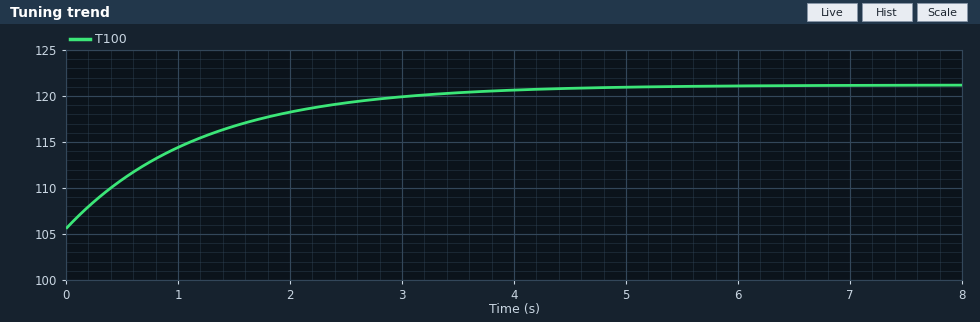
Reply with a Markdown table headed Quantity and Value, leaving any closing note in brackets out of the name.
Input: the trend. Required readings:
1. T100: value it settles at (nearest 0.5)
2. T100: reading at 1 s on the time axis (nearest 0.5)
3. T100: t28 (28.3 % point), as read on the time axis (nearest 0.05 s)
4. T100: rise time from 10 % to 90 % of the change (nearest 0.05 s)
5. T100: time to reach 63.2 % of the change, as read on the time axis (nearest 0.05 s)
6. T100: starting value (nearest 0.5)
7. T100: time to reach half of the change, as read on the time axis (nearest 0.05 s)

| Quantity | Value |
|---|---|
| T100: value it settles at | 121.0 |
| T100: reading at 1 s on the time axis | 114.5 |
| T100: t28 (28.3 % point), as read on the time axis | 0.40 s |
| T100: rise time from 10 % to 90 % of the change | 2.65 s |
| T100: time to reach 63.2 % of the change, as read on the time axis | 1.20 s |
| T100: starting value | 105.5 |
| T100: time to reach half of the change, as read on the time axis | 0.85 s |
